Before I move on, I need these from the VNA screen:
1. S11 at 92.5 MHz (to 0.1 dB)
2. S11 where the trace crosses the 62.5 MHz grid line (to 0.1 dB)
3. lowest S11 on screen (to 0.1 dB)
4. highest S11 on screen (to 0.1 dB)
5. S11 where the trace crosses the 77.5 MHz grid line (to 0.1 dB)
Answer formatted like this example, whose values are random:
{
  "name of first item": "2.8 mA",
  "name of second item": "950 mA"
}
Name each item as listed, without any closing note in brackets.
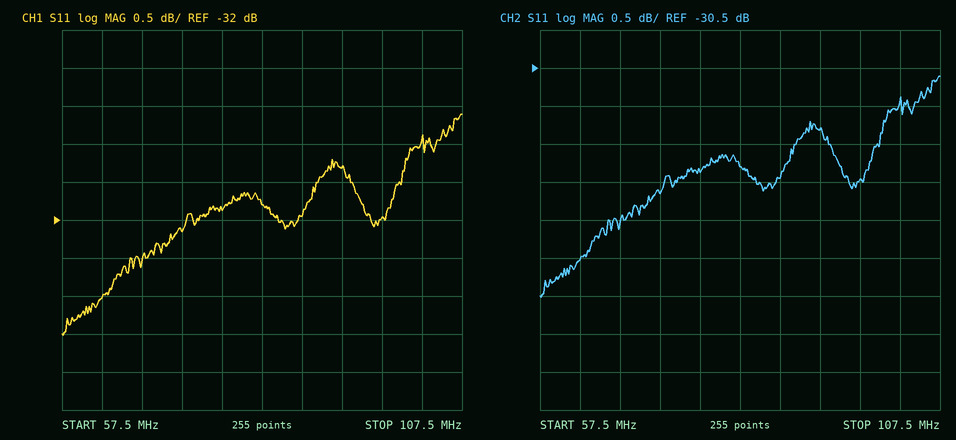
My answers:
{
  "S11 at 92.5 MHz": "-31.3 dB",
  "S11 where the trace crosses the 62.5 MHz grid line": "-33.0 dB",
  "lowest S11 on screen": "-33.5 dB",
  "highest S11 on screen": "-30.6 dB",
  "S11 where the trace crosses the 77.5 MHz grid line": "-31.9 dB"
}
